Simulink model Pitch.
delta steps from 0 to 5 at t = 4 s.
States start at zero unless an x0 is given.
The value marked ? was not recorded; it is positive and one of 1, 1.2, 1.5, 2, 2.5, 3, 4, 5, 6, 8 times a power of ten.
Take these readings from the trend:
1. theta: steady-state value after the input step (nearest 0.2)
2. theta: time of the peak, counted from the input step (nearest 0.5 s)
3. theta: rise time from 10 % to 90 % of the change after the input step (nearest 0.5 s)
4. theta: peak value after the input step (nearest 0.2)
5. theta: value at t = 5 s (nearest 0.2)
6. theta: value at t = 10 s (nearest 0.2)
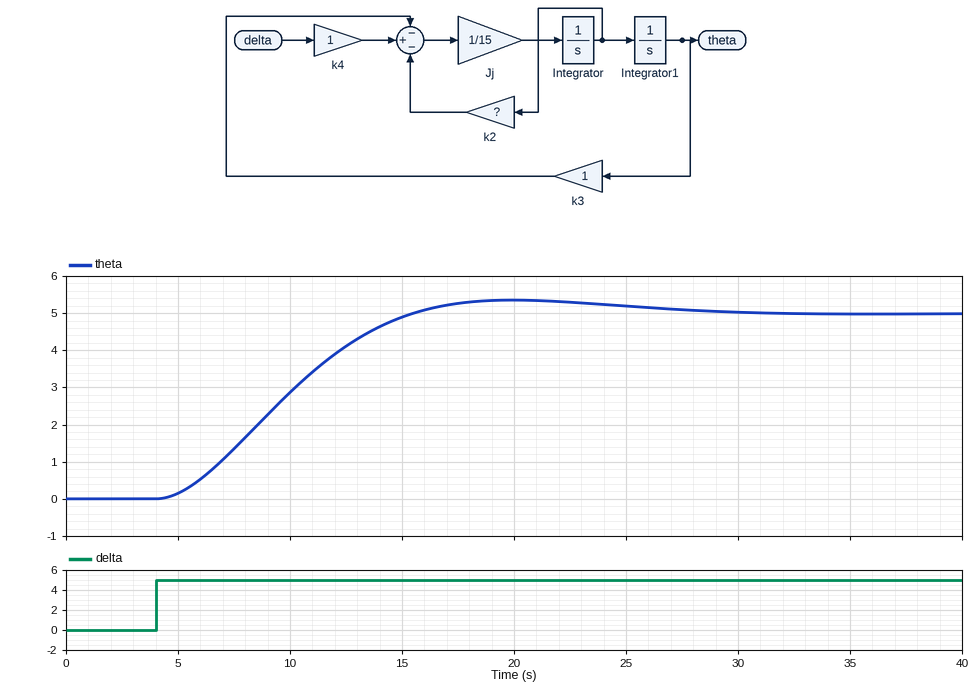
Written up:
5.0
16.0 s
7.5 s
5.4
0.2
2.8
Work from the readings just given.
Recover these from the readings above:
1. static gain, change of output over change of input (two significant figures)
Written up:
1.0
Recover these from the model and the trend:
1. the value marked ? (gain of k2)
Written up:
5
